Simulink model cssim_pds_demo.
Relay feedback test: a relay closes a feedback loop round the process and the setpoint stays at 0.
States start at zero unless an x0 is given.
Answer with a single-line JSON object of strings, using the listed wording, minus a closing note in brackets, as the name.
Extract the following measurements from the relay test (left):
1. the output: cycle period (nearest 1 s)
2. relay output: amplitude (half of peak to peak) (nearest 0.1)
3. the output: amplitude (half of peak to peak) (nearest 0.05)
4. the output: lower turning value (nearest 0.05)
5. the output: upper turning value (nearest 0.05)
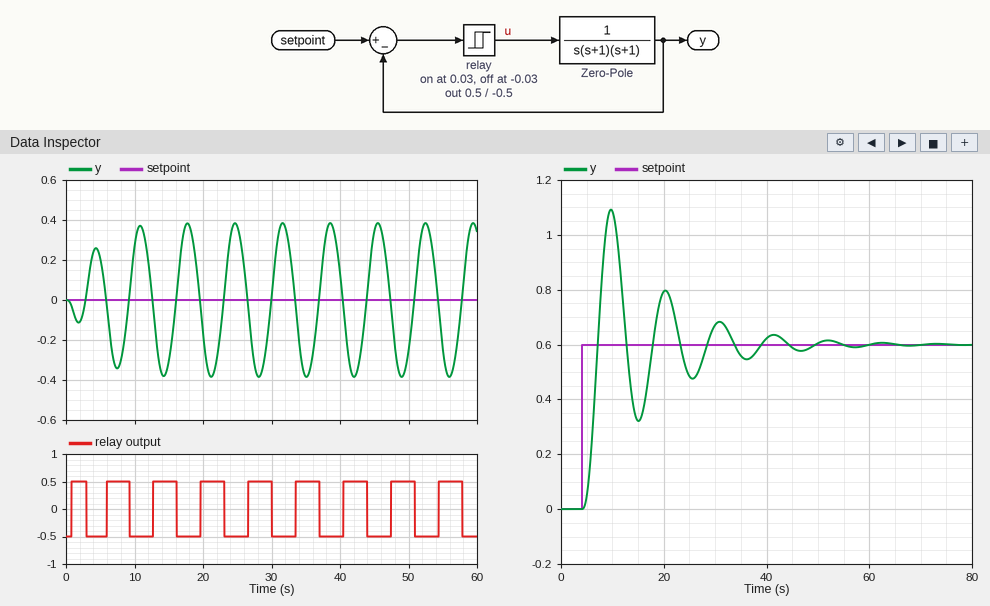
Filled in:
{"the output: cycle period": "7 s", "relay output: amplitude (half of peak to peak)": "0.5", "the output: amplitude (half of peak to peak)": "0.40", "the output: lower turning value": "-0.40", "the output: upper turning value": "0.40"}
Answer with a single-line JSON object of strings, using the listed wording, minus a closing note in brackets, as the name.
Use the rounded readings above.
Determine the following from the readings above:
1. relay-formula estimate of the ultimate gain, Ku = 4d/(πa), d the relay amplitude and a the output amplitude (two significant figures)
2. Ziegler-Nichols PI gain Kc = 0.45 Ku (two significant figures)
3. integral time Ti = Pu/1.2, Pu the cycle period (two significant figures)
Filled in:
{"relay-formula estimate of the ultimate gain, Ku = 4d/(πa), d the relay amplitude and a the output amplitude": "1.6", "Ziegler-Nichols PI gain Kc = 0.45 Ku": "0.72", "integral time Ti = Pu/1.2, Pu the cycle period": "5.8 s"}
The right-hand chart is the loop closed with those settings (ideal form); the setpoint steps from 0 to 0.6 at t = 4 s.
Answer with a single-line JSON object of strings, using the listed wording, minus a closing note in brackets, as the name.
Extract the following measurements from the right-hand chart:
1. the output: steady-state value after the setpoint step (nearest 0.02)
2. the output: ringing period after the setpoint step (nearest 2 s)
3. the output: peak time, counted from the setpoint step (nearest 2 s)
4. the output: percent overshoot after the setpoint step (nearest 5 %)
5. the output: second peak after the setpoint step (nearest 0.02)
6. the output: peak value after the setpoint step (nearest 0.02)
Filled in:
{"the output: steady-state value after the setpoint step": "0.60", "the output: ringing period after the setpoint step": "10 s", "the output: peak time, counted from the setpoint step": "6 s", "the output: percent overshoot after the setpoint step": "80 %", "the output: second peak after the setpoint step": "0.80", "the output: peak value after the setpoint step": "1.10"}
